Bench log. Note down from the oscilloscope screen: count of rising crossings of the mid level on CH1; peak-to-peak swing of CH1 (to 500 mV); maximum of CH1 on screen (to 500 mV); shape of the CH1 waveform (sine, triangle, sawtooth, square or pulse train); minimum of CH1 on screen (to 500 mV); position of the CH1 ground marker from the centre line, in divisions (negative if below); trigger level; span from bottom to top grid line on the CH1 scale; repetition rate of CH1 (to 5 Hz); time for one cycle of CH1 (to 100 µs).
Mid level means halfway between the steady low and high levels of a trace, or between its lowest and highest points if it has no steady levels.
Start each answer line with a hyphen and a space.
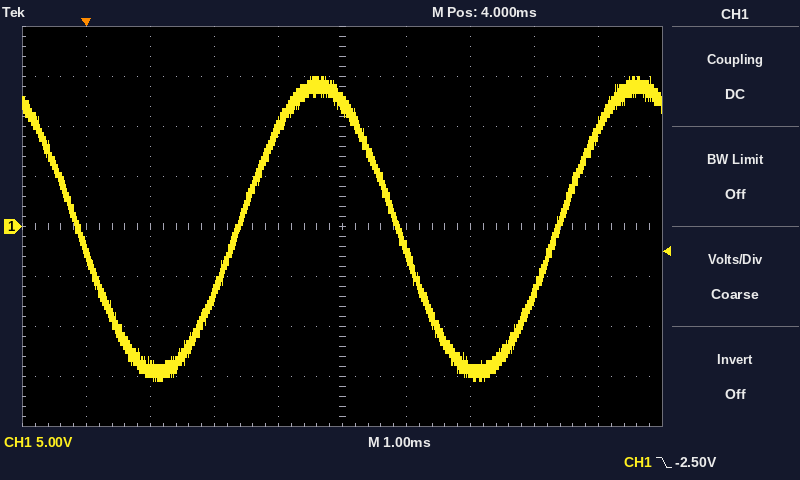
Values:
- 2
- 30.5 V
- 15.0 V
- sine
- -15.5 V
- 0.0 div
- -2.50 V
- 40 V
- 200 Hz
- 5.0 ms
